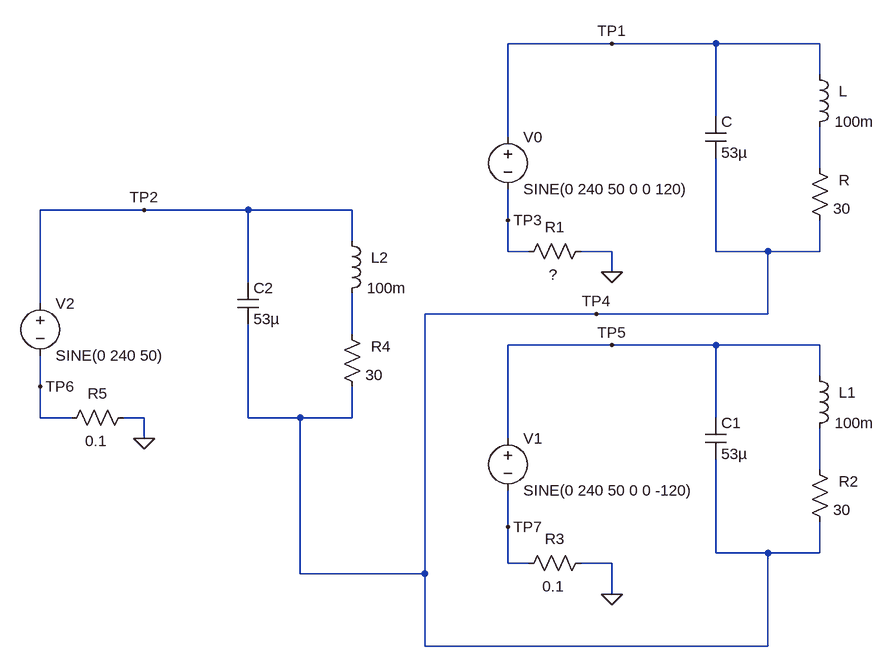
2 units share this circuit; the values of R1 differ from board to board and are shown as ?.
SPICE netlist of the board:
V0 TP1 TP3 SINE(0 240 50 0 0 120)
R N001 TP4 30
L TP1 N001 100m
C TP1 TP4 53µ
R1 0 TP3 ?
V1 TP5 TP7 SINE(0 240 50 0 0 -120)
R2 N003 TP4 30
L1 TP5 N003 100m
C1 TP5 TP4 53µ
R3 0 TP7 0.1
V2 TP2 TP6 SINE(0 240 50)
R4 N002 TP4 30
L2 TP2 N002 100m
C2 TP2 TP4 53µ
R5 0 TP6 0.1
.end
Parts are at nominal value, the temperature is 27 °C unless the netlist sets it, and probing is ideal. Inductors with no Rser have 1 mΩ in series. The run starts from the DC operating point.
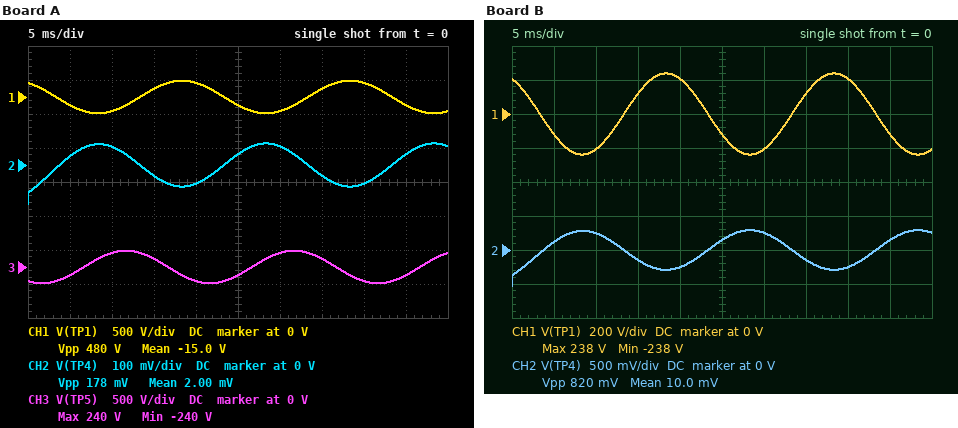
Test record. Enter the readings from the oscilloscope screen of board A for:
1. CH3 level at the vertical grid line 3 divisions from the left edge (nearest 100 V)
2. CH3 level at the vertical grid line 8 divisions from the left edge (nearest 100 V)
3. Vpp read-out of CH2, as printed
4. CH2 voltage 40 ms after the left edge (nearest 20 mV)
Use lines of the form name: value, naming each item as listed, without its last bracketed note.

CH3 level at the vertical grid line 3 divisions from the left edge: 100 V
CH3 level at the vertical grid line 8 divisions from the left edge: -200 V
Vpp read-out of CH2, as printed: 178 mV
CH2 voltage 40 ms after the left edge: -60 mV
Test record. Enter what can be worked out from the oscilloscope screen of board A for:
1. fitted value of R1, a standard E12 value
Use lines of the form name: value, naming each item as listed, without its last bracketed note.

fitted value of R1, a standard E12 value: 0.15 Ω
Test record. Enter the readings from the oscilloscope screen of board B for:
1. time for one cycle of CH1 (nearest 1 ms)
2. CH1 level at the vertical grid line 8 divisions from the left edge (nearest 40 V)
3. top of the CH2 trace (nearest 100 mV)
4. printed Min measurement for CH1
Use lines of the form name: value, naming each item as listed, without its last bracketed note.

time for one cycle of CH1: 20 ms
CH1 level at the vertical grid line 8 divisions from the left edge: 200 V
top of the CH2 trace: 300 mV
printed Min measurement for CH1: -238 V
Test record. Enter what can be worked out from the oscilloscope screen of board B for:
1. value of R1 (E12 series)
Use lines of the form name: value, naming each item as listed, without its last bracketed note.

value of R1: 0.33 Ω
